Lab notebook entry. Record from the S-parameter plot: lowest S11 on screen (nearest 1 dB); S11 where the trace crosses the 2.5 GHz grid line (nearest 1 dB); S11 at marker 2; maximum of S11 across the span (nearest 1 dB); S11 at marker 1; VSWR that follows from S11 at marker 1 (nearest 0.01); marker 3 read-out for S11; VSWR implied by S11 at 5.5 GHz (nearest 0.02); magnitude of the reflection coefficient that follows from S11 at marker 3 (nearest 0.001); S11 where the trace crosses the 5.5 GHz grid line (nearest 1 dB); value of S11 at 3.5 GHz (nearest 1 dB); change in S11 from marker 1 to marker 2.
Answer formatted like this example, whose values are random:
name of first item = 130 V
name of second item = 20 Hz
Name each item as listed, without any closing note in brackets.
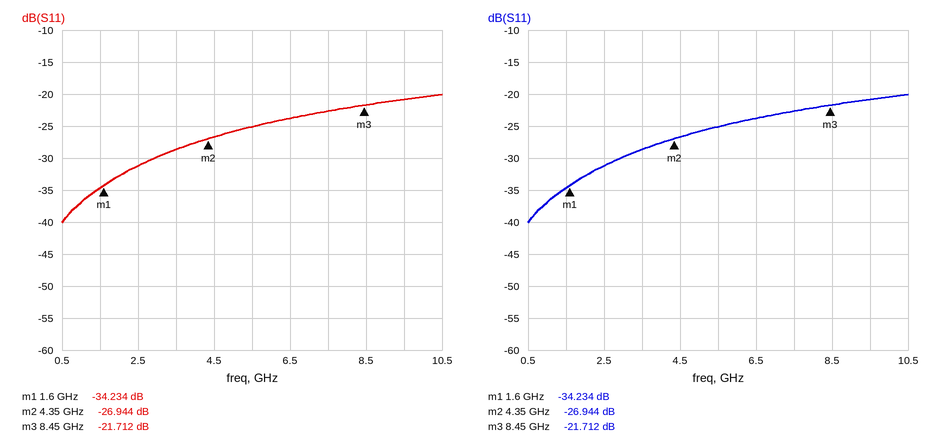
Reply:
lowest S11 on screen = -40 dB
S11 where the trace crosses the 2.5 GHz grid line = -31 dB
S11 at marker 2 = -26.944 dB
maximum of S11 across the span = -20 dB
S11 at marker 1 = -34.234 dB
VSWR that follows from S11 at marker 1 = 1.04
marker 3 read-out for S11 = -21.712 dB
VSWR implied by S11 at 5.5 GHz = 1.12
magnitude of the reflection coefficient that follows from S11 at marker 3 = 0.082
S11 where the trace crosses the 5.5 GHz grid line = -25 dB
value of S11 at 3.5 GHz = -29 dB
change in S11 from marker 1 to marker 2 = 7.290 dB
